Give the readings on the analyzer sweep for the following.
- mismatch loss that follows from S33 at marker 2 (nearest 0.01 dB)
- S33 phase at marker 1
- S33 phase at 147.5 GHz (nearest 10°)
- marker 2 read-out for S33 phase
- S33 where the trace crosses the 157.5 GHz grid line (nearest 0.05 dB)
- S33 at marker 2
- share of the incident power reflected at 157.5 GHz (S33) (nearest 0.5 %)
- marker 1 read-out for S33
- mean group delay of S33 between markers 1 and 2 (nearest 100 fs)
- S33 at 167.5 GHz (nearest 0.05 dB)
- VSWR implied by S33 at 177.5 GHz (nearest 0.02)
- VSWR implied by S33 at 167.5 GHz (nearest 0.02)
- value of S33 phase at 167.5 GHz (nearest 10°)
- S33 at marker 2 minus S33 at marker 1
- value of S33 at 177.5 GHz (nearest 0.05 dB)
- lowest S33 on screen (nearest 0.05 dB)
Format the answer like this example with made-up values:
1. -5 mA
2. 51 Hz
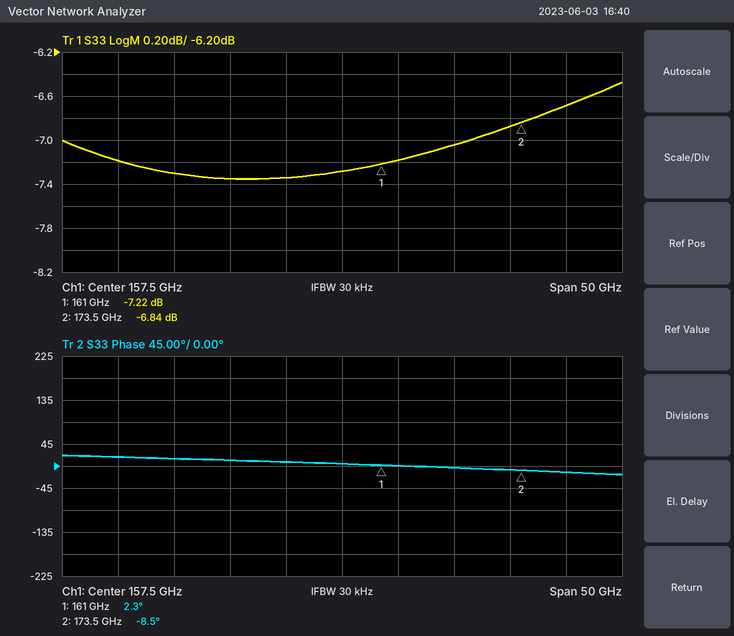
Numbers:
1. 1.01 dB
2. 2.3°
3. 10°
4. -8.5°
5. -7.30 dB
6. -6.84 dB
7. 18.5 %
8. -7.22 dB
9. 2.4 ps
10. -7.05 dB
11. 2.72
12. 2.60
13. 0°
14. 0.38 dB
15. -6.70 dB
16. -7.35 dB
